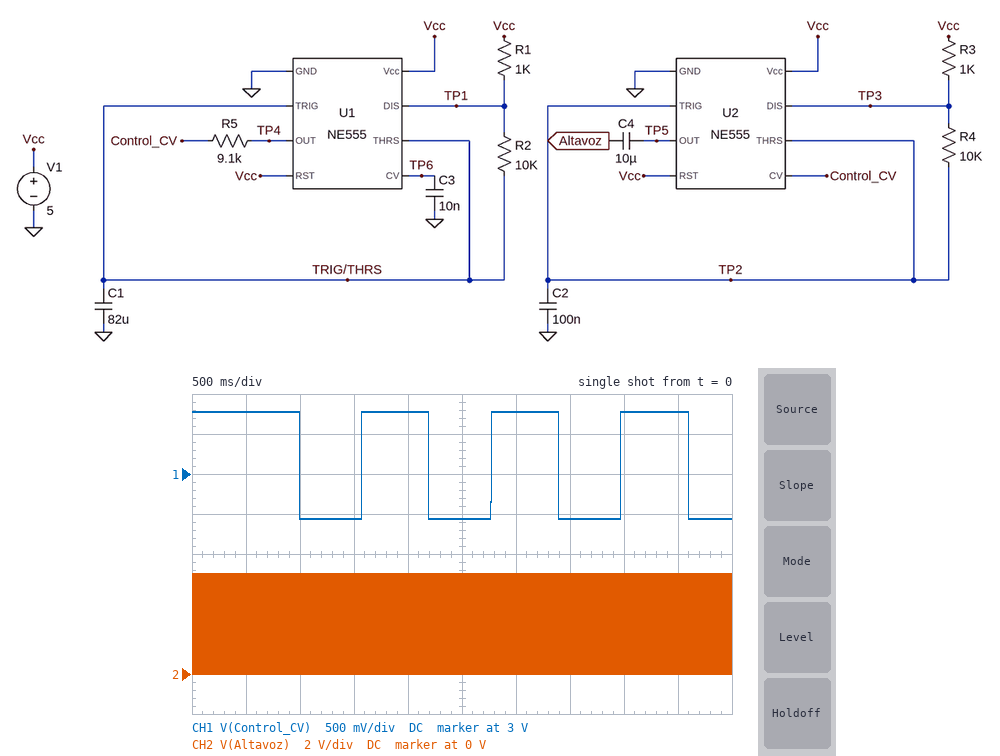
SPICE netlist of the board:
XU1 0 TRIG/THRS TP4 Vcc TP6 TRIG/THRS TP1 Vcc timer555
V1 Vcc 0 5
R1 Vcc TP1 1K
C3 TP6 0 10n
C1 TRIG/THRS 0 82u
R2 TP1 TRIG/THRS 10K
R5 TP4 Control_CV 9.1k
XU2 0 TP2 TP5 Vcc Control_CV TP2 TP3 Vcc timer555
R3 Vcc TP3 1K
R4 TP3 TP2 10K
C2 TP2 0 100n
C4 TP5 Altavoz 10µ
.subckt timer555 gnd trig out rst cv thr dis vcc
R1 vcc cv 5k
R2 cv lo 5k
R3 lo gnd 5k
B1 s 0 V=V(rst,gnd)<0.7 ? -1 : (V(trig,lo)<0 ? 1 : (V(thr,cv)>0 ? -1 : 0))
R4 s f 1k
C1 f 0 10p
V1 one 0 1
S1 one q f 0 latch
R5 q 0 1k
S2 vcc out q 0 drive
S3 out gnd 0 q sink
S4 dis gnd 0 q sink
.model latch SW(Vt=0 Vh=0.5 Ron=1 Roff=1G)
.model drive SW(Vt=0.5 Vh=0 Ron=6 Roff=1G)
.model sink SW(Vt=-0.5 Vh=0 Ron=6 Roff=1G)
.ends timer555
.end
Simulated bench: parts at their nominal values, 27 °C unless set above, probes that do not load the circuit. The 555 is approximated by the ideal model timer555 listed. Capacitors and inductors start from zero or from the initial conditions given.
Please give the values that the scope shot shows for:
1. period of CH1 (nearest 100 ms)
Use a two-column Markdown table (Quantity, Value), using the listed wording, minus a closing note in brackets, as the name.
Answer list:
| Quantity | Value |
|---|---|
| period of CH1 | 1.2 s |
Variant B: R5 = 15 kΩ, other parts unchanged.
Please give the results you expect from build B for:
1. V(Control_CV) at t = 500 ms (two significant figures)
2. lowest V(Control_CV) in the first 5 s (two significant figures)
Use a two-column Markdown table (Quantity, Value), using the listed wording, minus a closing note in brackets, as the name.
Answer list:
| Quantity | Value |
|---|---|
| V(Control_CV) at t = 500 ms | 3.6 V |
| lowest V(Control_CV) in the first 5 s | 2.7 V |
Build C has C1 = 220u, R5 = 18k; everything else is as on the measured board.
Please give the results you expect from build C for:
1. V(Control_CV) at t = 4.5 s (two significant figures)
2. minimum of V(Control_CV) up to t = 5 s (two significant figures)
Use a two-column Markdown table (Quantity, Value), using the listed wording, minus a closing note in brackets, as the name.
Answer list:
| Quantity | Value |
|---|---|
| V(Control_CV) at t = 4.5 s | 3.6 V |
| minimum of V(Control_CV) up to t = 5 s | 2.8 V |
